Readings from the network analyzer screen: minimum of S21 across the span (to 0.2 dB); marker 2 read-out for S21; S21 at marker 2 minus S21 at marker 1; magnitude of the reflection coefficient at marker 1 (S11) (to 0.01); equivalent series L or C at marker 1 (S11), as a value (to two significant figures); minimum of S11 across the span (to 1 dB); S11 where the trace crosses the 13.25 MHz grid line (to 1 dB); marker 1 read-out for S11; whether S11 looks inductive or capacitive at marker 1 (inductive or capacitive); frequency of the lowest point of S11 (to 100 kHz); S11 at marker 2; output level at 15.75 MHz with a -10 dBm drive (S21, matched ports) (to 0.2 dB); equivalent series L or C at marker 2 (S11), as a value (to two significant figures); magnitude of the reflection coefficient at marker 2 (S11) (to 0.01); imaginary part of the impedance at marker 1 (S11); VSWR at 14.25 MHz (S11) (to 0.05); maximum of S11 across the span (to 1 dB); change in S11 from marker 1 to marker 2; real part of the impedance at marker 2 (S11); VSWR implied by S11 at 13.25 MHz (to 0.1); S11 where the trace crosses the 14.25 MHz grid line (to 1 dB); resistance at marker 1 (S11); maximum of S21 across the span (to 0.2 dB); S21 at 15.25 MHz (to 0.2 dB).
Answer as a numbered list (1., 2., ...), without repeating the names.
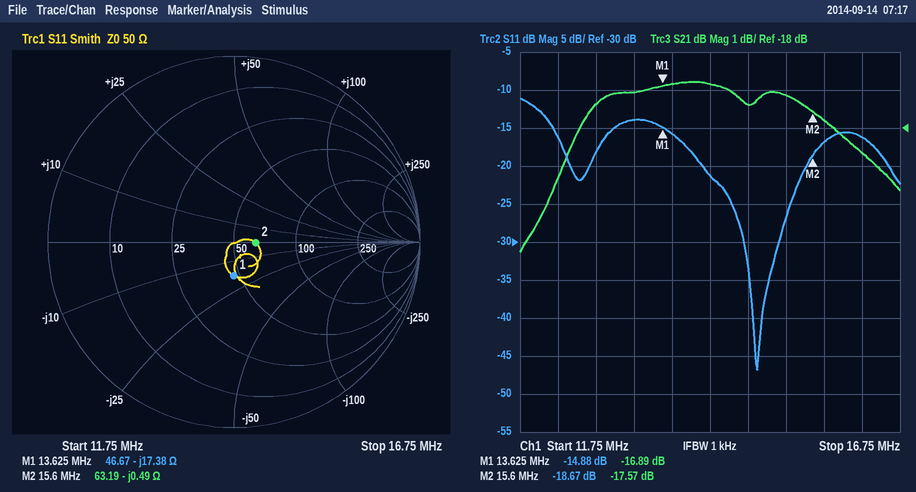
1. -21.2 dB
2. -17.57 dB
3. -0.68 dB
4. 0.18
5. 670 pF
6. -47 dB
7. -14 dB
8. -14.88 dB
9. capacitive
10. 14.9 MHz
11. -18.67 dB
12. -27.8 dBm
13. 21 nF
14. 0.12
15. -17.38 Ω
16. 1.20
17. -11 dB
18. -3.79 dB
19. 63.19 Ω
20. 1.5
21. -21 dB
22. 46.67 Ω
23. -16.8 dB
24. -17.2 dB
